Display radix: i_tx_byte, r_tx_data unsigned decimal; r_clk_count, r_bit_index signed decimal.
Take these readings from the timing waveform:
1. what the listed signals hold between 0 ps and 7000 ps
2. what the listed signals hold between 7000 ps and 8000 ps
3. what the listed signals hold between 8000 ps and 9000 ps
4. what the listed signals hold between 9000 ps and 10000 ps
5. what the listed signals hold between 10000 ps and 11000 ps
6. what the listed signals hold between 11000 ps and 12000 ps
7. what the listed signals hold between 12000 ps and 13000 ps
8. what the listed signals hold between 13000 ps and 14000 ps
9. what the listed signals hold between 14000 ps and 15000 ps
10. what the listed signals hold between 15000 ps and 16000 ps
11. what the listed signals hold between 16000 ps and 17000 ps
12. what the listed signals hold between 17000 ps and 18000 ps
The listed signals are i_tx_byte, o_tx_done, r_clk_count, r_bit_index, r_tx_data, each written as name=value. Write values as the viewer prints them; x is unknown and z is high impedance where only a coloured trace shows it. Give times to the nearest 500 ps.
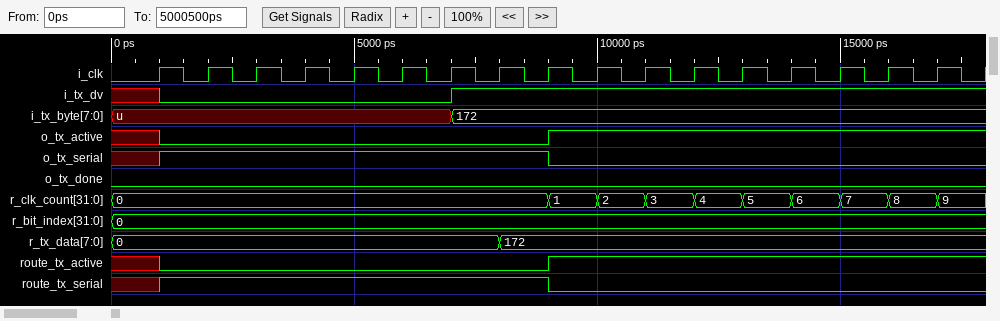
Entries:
i_tx_byte=u, o_tx_done=0, r_clk_count=0, r_bit_index=0, r_tx_data=0
i_tx_byte=172, o_tx_done=0, r_clk_count=0, r_bit_index=0, r_tx_data=0
i_tx_byte=172, o_tx_done=0, r_clk_count=0, r_bit_index=0, r_tx_data=172
i_tx_byte=172, o_tx_done=0, r_clk_count=1, r_bit_index=0, r_tx_data=172
i_tx_byte=172, o_tx_done=0, r_clk_count=2, r_bit_index=0, r_tx_data=172
i_tx_byte=172, o_tx_done=0, r_clk_count=3, r_bit_index=0, r_tx_data=172
i_tx_byte=172, o_tx_done=0, r_clk_count=4, r_bit_index=0, r_tx_data=172
i_tx_byte=172, o_tx_done=0, r_clk_count=5, r_bit_index=0, r_tx_data=172
i_tx_byte=172, o_tx_done=0, r_clk_count=6, r_bit_index=0, r_tx_data=172
i_tx_byte=172, o_tx_done=0, r_clk_count=7, r_bit_index=0, r_tx_data=172
i_tx_byte=172, o_tx_done=0, r_clk_count=8, r_bit_index=0, r_tx_data=172
i_tx_byte=172, o_tx_done=0, r_clk_count=9, r_bit_index=0, r_tx_data=172
